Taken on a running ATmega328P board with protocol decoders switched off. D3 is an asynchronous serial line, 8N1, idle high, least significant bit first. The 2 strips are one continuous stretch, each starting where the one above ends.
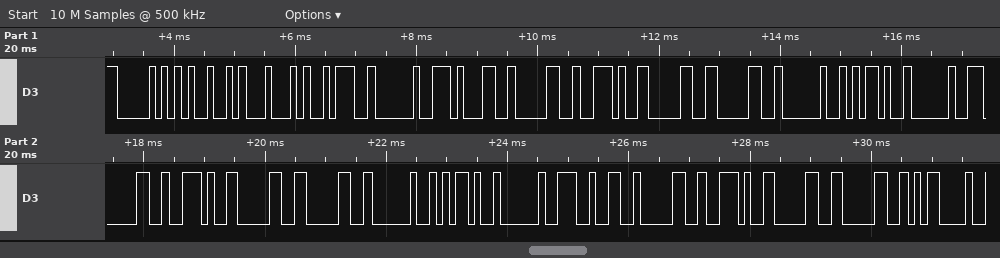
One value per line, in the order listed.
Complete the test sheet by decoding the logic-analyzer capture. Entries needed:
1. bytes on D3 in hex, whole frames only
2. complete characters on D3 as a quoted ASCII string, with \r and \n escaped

0x50 0x49 0x44 0x3A 0x20 0x31 0x30 0x2E 0x30 0x30 0x20 0x2D 0x20 0x30 0x2E 0x30 0x30 0x20 0x2D 0x20 0x32 0x30 0x2E 0x30 0x30 0x0D
"PID: 10.00 - 0.00 - 20.00\r"
